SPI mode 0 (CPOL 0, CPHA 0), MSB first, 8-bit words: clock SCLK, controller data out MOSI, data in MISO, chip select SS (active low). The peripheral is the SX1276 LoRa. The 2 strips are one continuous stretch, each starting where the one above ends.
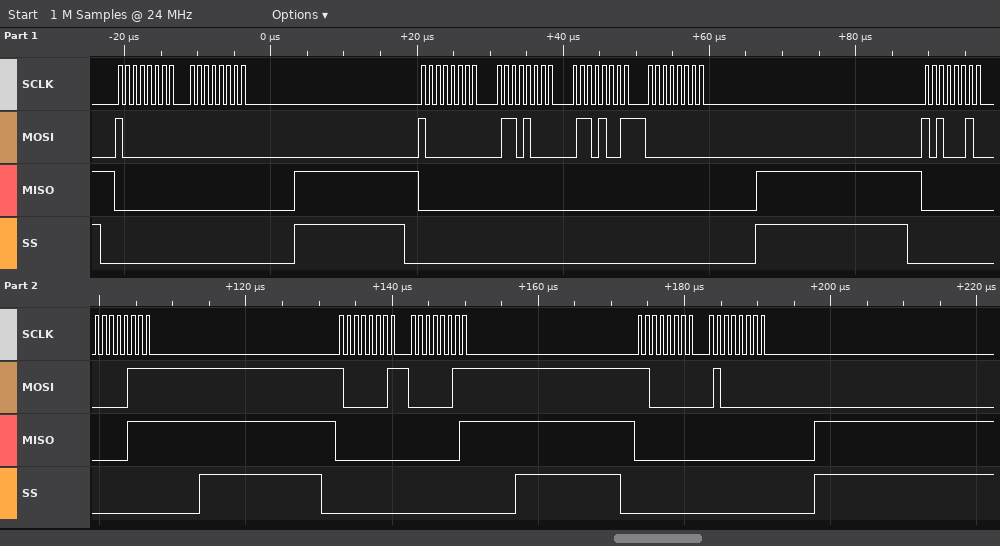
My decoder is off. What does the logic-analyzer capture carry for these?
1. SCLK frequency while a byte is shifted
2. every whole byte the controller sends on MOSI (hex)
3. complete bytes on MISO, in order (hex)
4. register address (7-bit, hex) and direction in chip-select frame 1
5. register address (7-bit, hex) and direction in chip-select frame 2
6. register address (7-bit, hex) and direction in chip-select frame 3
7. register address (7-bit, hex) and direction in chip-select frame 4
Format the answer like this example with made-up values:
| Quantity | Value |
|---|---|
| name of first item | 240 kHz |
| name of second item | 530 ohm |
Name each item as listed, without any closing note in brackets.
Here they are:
| Quantity | Value |
|---|---|
| SCLK frequency while a byte is shifted | 1 MHz |
| every whole byte the controller sends on MOSI | 0x80 0x00 0x80 0x68 0x69 0x00 0xA2 0x07 0x81 0x03 0xC0 0x40 |
| complete bytes on MISO, in order | 0x00 0x00 0x00 0x00 0x00 0x00 0x00 0x07 0x00 0x01 0x00 0x00 |
| register address (7-bit, hex) and direction in chip-select frame 1 | 0x00 write |
| register address (7-bit, hex) and direction in chip-select frame 2 | 0x00 write |
| register address (7-bit, hex) and direction in chip-select frame 3 | 0x22 write |
| register address (7-bit, hex) and direction in chip-select frame 4 | 0x01 write |
